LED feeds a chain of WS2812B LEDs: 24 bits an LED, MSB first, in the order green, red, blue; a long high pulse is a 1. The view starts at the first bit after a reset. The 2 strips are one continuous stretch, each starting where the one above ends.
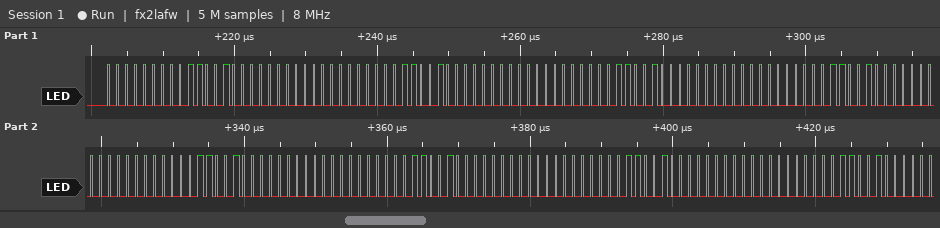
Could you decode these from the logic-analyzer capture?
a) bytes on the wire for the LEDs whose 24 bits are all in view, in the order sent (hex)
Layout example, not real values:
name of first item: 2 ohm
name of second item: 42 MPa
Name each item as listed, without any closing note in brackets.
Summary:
bytes on the wire for the LEDs whose 24 bits are all in view, in the order sent: 00 64 00 00 64 00 00 64 00 00 64 00 00 64 00 00 64 00 00 64 00
